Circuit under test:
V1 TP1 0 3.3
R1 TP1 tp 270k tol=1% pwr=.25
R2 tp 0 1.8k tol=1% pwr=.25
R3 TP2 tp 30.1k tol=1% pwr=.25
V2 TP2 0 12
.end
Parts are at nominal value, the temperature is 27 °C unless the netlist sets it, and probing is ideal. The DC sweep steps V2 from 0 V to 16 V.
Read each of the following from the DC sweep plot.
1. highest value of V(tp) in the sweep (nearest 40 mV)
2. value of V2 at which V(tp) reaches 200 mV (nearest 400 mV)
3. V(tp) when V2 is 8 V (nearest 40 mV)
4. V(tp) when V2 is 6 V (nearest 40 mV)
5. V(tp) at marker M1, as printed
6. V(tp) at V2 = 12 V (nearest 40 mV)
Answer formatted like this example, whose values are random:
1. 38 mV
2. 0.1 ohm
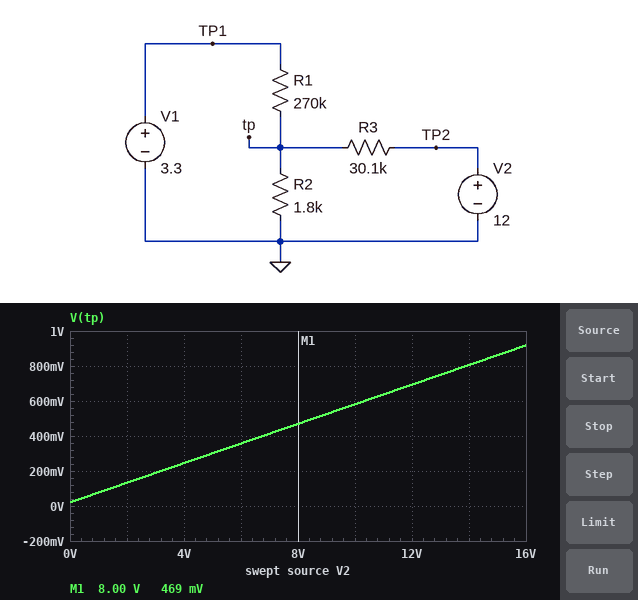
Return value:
1. 920 mV
2. 3.2 V
3. 480 mV
4. 360 mV
5. 469 mV
6. 680 mV
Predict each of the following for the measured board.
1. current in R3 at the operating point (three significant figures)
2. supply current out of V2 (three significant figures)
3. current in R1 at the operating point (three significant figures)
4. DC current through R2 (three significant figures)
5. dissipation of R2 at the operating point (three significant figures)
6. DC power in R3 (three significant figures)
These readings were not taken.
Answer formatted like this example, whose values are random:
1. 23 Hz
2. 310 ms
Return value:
1. 376 µA
2. 376 µA
3. 9.65 µA
4. 385 µA
5. 267 µW
6. 4.25 mW
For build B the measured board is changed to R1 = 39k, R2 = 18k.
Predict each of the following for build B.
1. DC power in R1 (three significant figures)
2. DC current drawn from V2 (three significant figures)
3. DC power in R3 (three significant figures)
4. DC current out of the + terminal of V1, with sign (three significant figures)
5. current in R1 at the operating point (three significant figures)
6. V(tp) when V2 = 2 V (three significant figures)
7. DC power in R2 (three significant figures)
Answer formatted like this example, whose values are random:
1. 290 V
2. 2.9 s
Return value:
1. 21.9 µW
2. 258 µA
3. 2.01 mW
4. -23.7 µA
5. 23.7 µA
6. 1.32 V
7. 991 µW
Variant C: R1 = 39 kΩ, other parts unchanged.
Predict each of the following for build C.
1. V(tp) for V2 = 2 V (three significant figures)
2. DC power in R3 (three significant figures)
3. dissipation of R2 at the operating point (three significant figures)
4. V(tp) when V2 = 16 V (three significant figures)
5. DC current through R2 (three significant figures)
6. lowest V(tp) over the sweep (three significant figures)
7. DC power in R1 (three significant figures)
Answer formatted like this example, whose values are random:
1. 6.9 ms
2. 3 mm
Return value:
1. 246 mV
2. 4.18 mW
3. 344 µW
4. 1.00 V
5. 437 µA
6. 138 mV
7. 162 µW
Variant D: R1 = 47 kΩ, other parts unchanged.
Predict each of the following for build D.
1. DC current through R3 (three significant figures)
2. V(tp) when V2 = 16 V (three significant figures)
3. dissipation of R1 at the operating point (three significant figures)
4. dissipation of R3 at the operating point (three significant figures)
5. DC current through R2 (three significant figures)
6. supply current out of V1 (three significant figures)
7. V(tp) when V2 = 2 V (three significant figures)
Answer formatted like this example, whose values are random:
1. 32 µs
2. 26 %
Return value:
1. 373 µA
2. 986 mV
3. 136 µW
4. 4.19 mW
5. 427 µA
6. 53.9 µA
7. 224 mV
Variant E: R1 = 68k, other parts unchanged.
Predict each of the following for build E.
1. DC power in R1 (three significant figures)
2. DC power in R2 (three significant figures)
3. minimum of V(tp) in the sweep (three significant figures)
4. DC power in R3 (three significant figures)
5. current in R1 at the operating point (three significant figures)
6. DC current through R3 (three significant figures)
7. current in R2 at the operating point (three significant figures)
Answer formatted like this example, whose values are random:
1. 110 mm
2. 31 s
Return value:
1. 96.3 µW
2. 305 µW
3. 80.4 mV
4. 4.21 mW
5. 37.6 µA
6. 374 µA
7. 412 µA
